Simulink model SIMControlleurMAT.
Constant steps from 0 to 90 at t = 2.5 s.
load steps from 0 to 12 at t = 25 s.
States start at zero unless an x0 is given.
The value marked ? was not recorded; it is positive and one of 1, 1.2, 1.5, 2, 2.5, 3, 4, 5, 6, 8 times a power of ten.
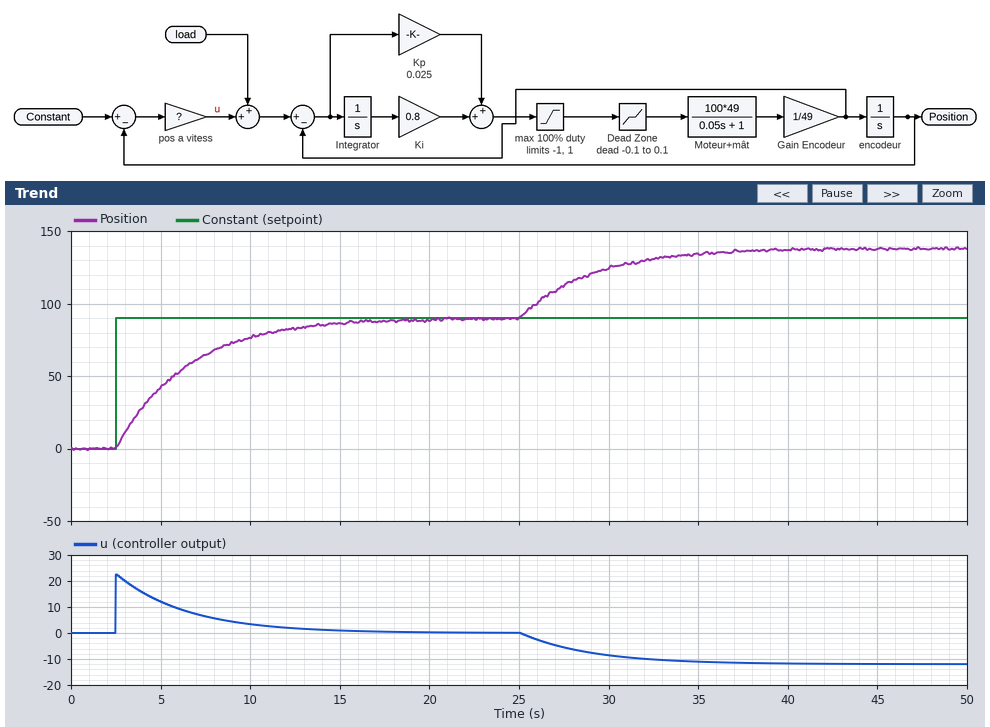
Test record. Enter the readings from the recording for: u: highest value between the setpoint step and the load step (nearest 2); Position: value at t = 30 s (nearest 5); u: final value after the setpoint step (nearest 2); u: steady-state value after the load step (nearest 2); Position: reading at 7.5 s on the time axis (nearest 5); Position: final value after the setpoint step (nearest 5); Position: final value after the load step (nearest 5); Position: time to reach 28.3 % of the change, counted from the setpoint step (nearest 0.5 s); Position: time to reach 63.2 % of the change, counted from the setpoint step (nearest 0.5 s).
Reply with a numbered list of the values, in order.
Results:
1. 22
2. 125
3. 0
4. -12
5. 65
6. 90
7. 140
8. 1.5 s
9. 4.0 s
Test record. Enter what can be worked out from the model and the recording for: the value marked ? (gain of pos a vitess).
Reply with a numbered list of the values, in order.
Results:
1. 0.25
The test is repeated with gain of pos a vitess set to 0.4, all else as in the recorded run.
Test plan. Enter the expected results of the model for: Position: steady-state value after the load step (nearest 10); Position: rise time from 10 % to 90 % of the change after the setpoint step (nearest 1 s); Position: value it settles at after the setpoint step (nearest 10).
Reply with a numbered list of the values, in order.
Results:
1. 120
2. 5 s
3. 90
